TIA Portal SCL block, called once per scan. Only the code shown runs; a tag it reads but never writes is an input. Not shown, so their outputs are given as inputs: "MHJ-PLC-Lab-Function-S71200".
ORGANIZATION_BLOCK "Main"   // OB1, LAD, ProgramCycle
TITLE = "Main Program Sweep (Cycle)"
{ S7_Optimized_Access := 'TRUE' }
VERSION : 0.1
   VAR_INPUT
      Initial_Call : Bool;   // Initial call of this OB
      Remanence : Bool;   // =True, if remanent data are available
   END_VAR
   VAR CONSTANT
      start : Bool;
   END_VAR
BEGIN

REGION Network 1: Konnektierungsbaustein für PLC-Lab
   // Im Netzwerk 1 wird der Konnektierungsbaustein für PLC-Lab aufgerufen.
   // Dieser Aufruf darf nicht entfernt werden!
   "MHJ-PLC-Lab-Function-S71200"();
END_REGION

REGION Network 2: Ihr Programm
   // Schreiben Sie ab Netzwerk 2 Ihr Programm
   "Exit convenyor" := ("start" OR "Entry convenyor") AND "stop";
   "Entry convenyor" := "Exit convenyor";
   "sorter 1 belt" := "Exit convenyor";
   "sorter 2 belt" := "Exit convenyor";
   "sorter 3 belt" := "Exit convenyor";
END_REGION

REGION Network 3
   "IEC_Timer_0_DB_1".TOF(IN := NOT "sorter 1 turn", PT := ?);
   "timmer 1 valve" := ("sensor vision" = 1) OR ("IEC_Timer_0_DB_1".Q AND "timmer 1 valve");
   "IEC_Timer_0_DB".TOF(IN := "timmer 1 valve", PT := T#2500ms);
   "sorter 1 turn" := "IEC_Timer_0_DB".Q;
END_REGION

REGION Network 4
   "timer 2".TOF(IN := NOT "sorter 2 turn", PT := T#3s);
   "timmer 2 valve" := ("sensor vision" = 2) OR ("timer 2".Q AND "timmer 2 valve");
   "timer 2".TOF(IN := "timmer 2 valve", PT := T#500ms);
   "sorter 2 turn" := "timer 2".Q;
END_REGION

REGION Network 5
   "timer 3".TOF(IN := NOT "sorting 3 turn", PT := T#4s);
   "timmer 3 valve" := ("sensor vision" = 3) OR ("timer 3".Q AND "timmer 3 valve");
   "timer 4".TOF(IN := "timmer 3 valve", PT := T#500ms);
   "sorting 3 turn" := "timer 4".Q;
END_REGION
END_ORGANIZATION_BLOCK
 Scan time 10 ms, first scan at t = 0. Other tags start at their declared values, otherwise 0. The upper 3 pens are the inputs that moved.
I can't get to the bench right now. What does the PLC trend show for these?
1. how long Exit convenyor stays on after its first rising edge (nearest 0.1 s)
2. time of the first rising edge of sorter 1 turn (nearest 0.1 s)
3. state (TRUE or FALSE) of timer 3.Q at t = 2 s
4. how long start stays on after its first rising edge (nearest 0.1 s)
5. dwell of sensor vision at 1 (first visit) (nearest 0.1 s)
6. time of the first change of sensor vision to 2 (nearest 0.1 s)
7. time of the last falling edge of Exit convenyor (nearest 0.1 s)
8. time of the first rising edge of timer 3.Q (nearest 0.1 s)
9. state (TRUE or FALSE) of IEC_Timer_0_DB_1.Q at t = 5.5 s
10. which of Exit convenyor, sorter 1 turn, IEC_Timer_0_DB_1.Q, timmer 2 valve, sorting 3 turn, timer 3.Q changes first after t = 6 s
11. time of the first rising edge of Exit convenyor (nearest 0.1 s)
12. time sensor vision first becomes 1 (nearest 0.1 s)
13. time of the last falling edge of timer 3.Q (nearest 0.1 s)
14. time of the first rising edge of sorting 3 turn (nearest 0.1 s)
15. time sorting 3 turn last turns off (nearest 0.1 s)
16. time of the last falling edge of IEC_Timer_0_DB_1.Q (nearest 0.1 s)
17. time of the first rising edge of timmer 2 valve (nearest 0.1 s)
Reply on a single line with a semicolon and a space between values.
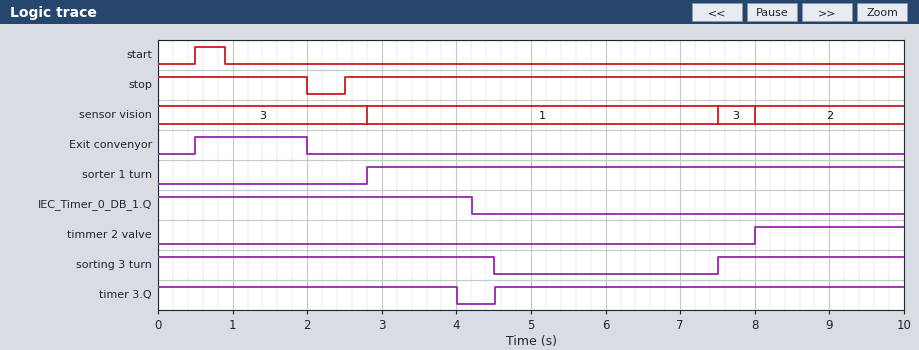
1.5 s; 2.8 s; TRUE; 0.4 s; 4.7 s; 8.0 s; 2.0 s; 4.5 s; FALSE; sorting 3 turn; 0.5 s; 2.8 s; 4.0 s; 7.5 s; 4.5 s; 4.2 s; 8.0 s
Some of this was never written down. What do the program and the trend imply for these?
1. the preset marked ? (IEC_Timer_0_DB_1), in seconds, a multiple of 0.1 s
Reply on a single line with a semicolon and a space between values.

1.4 s
